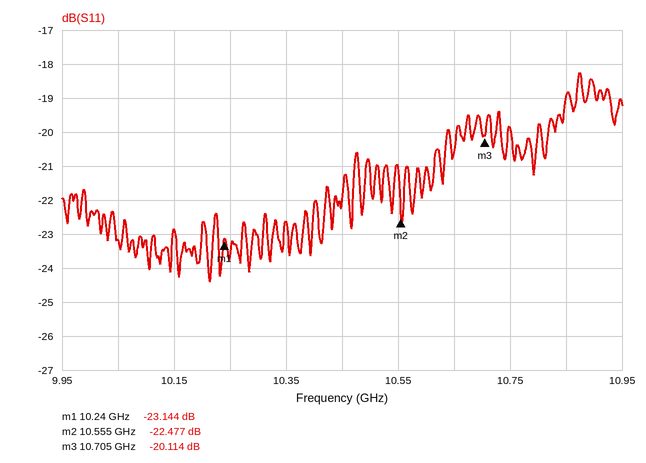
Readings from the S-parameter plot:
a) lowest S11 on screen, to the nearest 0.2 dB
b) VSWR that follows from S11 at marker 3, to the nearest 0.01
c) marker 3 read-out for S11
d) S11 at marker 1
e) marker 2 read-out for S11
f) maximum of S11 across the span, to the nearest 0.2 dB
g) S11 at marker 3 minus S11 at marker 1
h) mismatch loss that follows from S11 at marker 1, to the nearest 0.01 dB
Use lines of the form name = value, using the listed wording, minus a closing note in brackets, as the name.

lowest S11 on screen, to the nearest 0.2 dB = -24.4 dB
VSWR that follows from S11 at marker 3, to the nearest 0.01 = 1.22
marker 3 read-out for S11 = -20.114 dB
S11 at marker 1 = -23.144 dB
marker 2 read-out for S11 = -22.477 dB
maximum of S11 across the span, to the nearest 0.2 dB = -18.2 dB
S11 at marker 3 minus S11 at marker 1 = 3.030 dB
mismatch loss that follows from S11 at marker 1, to the nearest 0.01 dB = 0.02 dB
